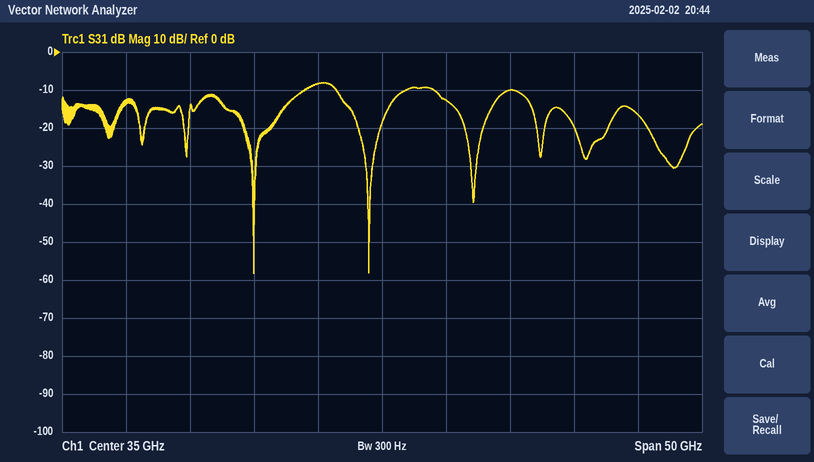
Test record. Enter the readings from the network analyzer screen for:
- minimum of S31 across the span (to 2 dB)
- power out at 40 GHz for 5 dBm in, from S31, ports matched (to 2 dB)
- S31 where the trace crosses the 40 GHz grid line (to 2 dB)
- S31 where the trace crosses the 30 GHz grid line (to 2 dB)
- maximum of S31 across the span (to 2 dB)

-58 dB
-8 dBm
-12 dB
-8 dB
-8 dB
